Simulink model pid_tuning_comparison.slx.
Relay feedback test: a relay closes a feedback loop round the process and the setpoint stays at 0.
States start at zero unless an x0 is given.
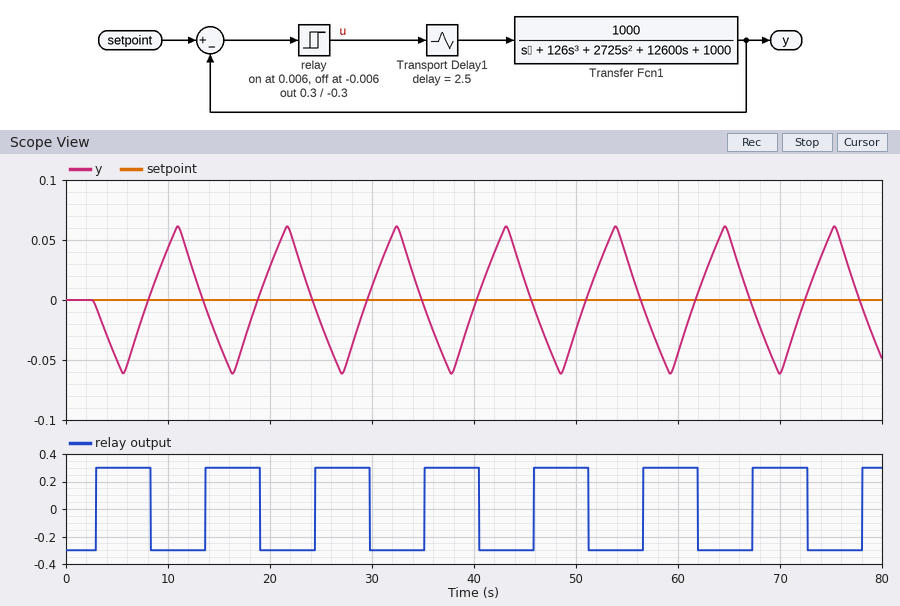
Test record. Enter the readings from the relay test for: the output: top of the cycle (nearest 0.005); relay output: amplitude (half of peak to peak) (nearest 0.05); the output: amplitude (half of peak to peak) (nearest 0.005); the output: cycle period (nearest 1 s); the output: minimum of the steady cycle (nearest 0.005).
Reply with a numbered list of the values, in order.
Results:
1. 0.060
2. 0.30
3. 0.060
4. 11 s
5. -0.060
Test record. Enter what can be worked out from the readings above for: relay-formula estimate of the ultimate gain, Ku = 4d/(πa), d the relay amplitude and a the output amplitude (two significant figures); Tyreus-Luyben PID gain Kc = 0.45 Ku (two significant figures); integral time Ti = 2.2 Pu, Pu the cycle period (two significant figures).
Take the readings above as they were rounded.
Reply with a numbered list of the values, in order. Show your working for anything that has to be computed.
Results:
1. 4 × 0.3 / (π × 0.06) = 6.4
2. 0.45 × 6.4 = 2.9
3. 2.2 × 11 = 24 s
